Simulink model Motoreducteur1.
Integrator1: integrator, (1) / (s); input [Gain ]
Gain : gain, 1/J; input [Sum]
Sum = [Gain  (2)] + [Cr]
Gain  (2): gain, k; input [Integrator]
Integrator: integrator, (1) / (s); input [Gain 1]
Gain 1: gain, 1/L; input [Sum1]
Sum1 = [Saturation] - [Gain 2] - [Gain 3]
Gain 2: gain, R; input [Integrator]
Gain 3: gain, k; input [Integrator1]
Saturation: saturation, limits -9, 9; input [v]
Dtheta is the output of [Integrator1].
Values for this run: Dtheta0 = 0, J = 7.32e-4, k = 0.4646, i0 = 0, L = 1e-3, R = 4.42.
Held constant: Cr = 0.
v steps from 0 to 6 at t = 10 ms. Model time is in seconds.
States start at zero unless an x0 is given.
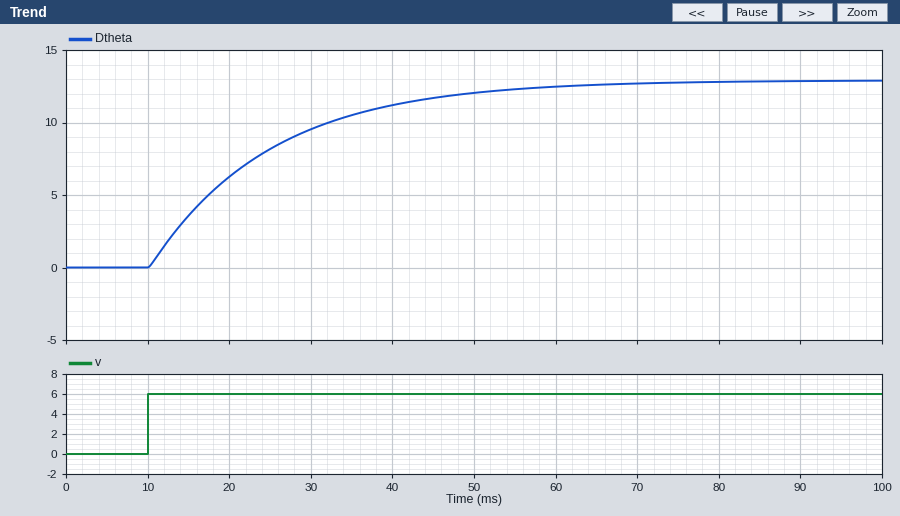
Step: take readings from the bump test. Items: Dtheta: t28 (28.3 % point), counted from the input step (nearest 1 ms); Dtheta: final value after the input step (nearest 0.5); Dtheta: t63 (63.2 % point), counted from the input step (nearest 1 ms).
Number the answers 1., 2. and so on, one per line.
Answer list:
1. 5 ms
2. 13.0
3. 15 ms
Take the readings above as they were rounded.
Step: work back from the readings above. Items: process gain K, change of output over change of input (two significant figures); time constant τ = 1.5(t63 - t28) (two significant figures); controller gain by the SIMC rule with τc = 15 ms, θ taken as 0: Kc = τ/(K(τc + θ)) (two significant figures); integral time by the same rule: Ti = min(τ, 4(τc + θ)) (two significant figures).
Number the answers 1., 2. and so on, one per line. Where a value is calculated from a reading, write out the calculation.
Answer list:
1. (13 - 0) / 6 = 2.2
2. 1.5 × (15 - 5) = 15 ms
3. 15 / (2.2 × (15 + 0)) = 0.45
4. min(15, 4 × (15 + 0)) = 15 ms
